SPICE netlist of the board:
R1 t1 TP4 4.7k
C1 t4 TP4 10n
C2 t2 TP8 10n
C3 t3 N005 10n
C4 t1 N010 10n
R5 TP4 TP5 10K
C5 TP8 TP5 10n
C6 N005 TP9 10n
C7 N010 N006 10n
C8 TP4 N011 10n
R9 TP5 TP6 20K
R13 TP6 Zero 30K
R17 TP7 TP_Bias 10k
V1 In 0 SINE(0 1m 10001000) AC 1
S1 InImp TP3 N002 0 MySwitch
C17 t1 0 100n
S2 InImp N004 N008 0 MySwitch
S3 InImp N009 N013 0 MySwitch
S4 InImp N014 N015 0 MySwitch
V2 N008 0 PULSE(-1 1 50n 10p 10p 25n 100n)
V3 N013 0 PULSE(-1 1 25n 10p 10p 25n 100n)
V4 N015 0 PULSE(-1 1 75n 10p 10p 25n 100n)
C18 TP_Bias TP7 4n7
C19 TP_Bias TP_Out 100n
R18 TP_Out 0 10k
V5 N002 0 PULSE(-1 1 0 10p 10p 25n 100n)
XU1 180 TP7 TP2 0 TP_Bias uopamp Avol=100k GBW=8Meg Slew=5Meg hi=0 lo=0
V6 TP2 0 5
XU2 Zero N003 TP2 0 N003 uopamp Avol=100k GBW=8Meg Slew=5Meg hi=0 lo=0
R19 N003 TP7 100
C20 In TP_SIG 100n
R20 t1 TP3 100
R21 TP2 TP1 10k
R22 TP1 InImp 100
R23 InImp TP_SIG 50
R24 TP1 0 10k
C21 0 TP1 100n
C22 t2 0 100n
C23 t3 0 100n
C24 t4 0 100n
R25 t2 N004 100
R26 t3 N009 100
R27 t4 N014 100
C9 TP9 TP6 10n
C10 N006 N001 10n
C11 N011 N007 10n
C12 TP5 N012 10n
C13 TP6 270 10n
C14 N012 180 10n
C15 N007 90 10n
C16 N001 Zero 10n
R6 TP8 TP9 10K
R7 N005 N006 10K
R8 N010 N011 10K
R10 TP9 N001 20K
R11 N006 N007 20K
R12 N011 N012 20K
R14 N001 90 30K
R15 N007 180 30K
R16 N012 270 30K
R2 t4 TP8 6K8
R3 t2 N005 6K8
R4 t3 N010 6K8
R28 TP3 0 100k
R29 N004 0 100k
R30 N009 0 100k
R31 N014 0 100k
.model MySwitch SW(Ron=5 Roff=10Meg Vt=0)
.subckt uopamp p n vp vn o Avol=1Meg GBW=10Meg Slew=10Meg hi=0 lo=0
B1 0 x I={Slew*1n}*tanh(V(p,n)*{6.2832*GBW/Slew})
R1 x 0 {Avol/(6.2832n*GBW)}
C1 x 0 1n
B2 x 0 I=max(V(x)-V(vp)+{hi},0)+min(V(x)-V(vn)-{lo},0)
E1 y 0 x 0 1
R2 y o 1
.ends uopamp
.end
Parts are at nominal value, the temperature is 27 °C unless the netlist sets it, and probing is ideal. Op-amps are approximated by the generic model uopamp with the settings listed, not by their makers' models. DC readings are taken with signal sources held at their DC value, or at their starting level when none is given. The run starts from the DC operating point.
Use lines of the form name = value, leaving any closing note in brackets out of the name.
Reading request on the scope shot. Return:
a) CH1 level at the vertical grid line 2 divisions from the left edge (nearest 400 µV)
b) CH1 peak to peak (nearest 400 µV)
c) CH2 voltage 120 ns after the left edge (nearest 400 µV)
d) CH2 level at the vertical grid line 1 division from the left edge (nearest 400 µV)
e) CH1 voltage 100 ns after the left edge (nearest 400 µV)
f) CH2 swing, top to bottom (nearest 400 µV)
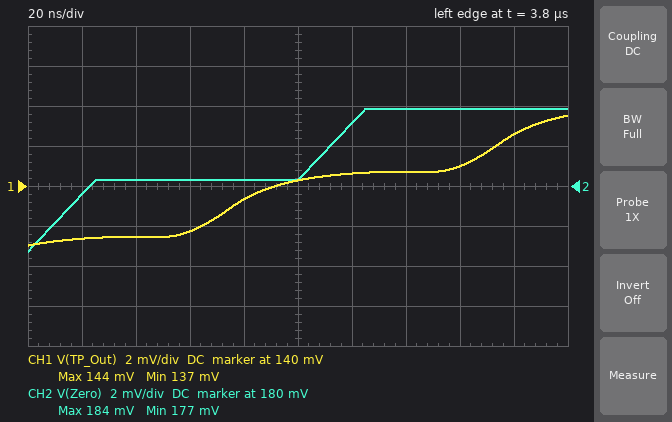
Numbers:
CH1 level at the vertical grid line 2 divisions from the left edge = 137.6 mV
CH1 peak to peak = 6.4 mV
CH2 voltage 120 ns after the left edge = 183.2 mV
CH2 level at the vertical grid line 1 division from the left edge = 179.6 mV
CH1 voltage 100 ns after the left edge = 140.4 mV
CH2 swing, top to bottom = 7.2 mV
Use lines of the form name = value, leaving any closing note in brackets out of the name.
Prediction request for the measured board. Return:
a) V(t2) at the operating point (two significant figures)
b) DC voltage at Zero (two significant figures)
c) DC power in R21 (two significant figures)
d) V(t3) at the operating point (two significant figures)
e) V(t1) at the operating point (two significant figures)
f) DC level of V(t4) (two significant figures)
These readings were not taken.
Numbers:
V(t2) at the operating point = 25 mV
DC voltage at Zero = 25 mV
DC power in R21 = 630 µW
V(t3) at the operating point = 25 mV
V(t1) at the operating point = 25 mV
DC level of V(t4) = 25 mV
